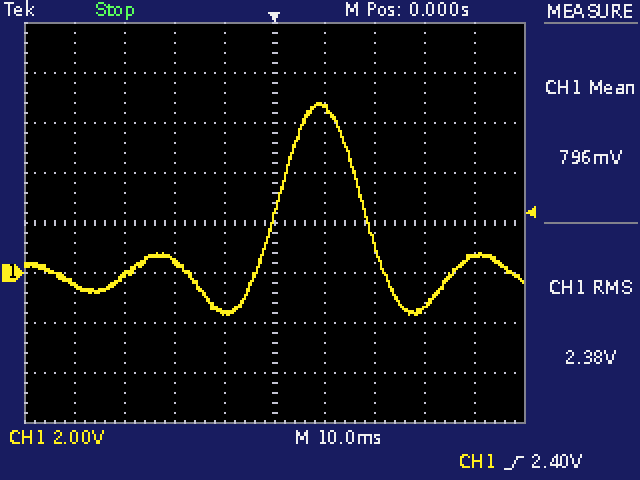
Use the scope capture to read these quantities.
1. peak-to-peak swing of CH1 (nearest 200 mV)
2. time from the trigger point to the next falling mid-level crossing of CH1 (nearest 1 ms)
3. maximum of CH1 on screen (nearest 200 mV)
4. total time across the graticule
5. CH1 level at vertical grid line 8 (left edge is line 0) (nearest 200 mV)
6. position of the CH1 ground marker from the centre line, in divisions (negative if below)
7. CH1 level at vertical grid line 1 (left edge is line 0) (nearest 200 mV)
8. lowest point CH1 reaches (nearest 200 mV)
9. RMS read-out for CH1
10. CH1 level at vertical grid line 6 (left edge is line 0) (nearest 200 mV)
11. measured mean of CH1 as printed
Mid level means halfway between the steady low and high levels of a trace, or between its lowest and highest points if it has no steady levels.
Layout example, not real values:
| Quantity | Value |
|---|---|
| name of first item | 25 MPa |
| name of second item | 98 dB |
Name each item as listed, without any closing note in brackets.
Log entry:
| Quantity | Value |
|---|---|
| peak-to-peak swing of CH1 | 8.4 V |
| time from the trigger point to the next falling mid-level crossing of CH1 | 18 ms |
| maximum of CH1 on screen | 6.8 V |
| total time across the graticule | 100 ms |
| CH1 level at vertical grid line 8 (left edge is line 0) | -1.4 V |
| position of the CH1 ground marker from the centre line, in divisions | -1.0 div |
| CH1 level at vertical grid line 1 (left edge is line 0) | -400 mV |
| lowest point CH1 reaches | -1.6 V |
| RMS read-out for CH1 | 2.38 V |
| CH1 level at vertical grid line 6 (left edge is line 0) | 6.6 V |
| measured mean of CH1 as printed | 796 mV |
